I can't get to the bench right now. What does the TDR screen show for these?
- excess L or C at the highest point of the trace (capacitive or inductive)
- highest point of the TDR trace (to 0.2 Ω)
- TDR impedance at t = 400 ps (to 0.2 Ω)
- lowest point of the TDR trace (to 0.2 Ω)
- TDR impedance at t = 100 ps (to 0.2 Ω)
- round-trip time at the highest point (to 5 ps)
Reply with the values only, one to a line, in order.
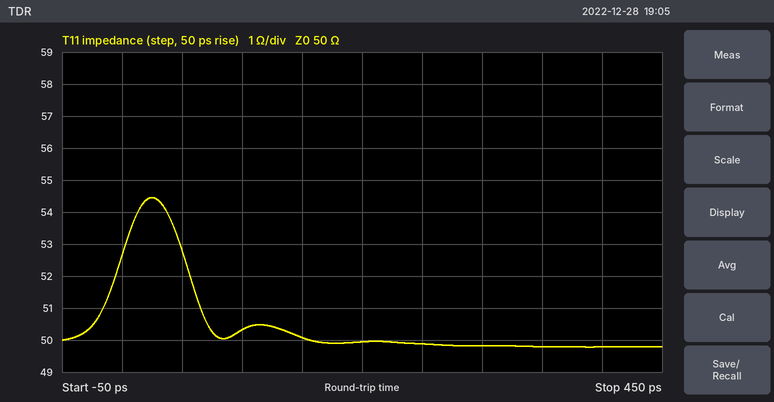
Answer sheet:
inductive
54.4 Ω
49.8 Ω
49.8 Ω
50.4 Ω
25 ps
